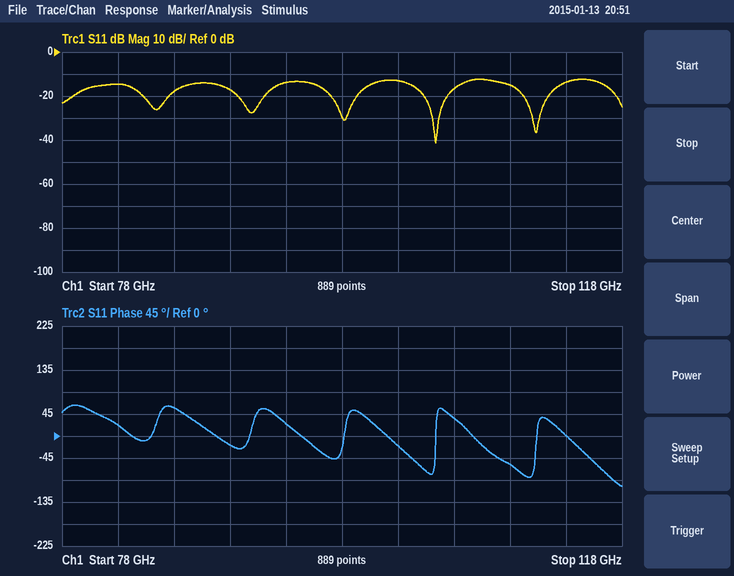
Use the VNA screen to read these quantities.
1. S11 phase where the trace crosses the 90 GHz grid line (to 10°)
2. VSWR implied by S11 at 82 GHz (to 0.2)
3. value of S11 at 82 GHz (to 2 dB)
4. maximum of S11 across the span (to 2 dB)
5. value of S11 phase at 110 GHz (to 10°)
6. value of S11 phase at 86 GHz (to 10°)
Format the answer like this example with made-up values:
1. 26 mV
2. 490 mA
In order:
1. -20°
2. 1.4
3. -14 dB
4. -12 dB
5. -60°
6. 60°
